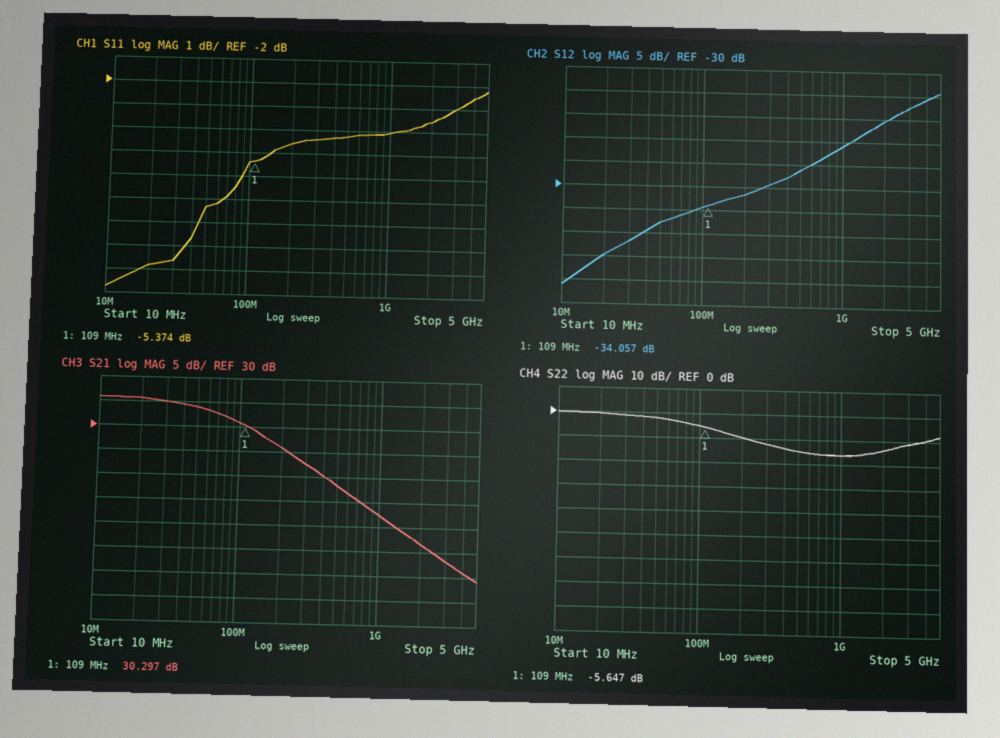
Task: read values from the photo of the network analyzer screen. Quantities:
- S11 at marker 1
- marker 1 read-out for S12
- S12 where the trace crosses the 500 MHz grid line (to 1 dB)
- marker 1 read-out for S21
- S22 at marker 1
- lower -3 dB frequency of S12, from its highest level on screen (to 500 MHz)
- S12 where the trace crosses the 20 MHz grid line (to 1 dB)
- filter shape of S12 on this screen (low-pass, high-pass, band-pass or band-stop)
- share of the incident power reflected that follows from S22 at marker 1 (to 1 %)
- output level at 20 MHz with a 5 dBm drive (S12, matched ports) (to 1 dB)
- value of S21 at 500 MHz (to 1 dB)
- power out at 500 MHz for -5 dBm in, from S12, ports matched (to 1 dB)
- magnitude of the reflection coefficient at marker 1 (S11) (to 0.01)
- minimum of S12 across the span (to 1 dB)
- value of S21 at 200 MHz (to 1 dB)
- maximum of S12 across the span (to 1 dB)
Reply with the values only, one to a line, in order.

-5.374 dB
-34.057 dB
-26 dB
30.297 dB
-5.647 dB
3.0 GHz
-45 dB
high-pass
27 %
-40 dBm
18 dB
-31 dBm
0.54
-51 dB
26 dB
-9 dB
